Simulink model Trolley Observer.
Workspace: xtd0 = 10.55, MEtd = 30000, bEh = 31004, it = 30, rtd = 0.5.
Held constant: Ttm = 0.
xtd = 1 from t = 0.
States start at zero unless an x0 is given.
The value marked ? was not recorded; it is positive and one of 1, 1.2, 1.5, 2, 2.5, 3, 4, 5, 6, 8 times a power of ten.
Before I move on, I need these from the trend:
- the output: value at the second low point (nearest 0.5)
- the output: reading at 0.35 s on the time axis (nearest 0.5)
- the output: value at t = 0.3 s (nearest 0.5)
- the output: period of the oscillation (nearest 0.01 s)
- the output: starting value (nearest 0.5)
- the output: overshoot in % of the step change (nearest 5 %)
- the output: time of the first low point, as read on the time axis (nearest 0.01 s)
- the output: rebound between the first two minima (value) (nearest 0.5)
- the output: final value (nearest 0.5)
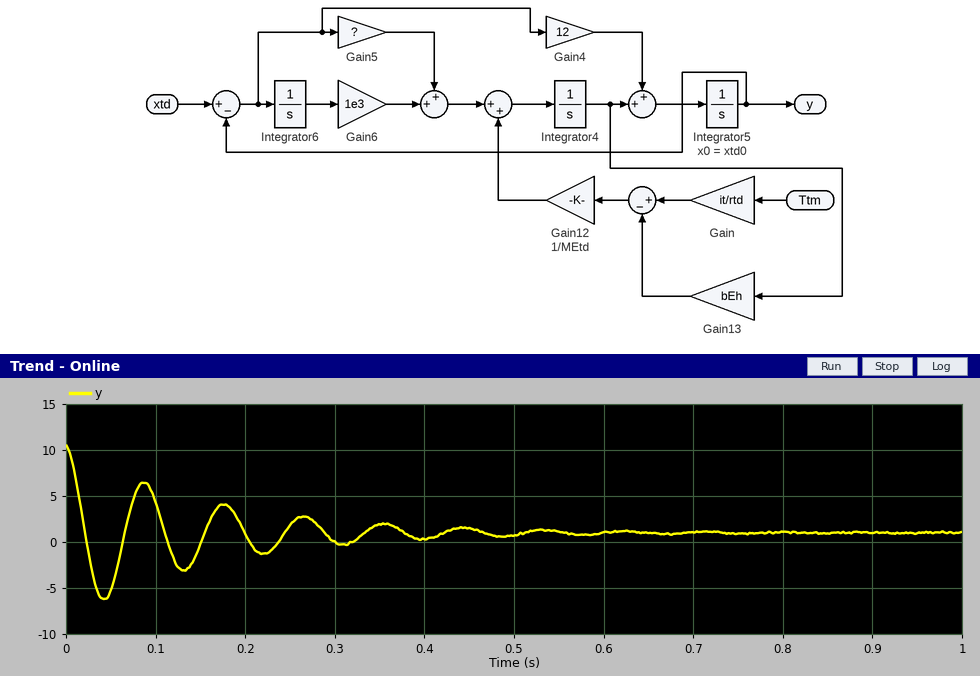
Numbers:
-3.0
2.0
0.0
0.09 s
10.5
75 %
0.04 s
6.5
1.0
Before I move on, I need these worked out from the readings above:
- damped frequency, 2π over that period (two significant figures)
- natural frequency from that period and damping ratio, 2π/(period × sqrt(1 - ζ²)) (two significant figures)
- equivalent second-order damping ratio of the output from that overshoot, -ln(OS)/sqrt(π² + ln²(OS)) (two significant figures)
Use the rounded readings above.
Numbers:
70 rad/s
70 rad/s
0.091
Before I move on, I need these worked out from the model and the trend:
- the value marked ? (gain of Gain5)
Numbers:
5000
